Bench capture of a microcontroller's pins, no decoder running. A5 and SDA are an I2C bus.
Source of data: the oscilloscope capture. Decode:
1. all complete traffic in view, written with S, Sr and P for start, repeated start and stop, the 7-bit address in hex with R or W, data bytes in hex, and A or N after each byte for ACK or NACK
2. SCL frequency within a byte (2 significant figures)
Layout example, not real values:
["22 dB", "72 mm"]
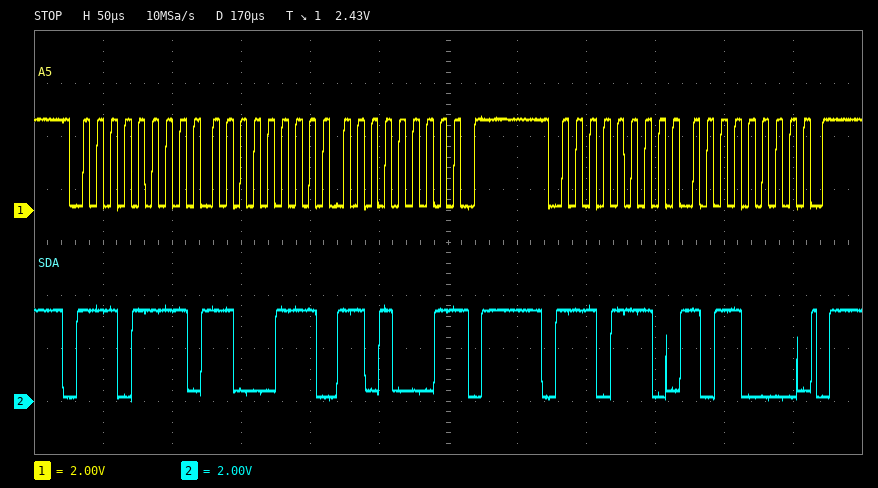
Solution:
["S 77R A C7 A D1 N P S 77W A B0 A P", "100 kHz"]
